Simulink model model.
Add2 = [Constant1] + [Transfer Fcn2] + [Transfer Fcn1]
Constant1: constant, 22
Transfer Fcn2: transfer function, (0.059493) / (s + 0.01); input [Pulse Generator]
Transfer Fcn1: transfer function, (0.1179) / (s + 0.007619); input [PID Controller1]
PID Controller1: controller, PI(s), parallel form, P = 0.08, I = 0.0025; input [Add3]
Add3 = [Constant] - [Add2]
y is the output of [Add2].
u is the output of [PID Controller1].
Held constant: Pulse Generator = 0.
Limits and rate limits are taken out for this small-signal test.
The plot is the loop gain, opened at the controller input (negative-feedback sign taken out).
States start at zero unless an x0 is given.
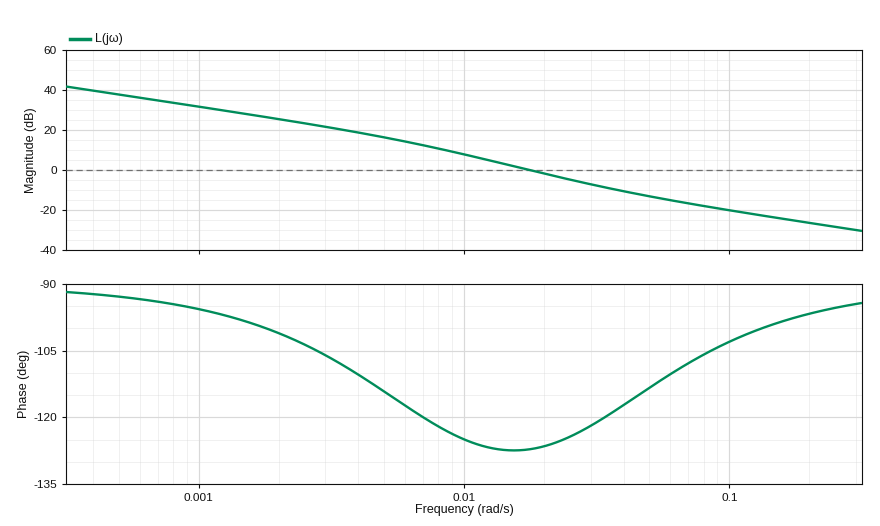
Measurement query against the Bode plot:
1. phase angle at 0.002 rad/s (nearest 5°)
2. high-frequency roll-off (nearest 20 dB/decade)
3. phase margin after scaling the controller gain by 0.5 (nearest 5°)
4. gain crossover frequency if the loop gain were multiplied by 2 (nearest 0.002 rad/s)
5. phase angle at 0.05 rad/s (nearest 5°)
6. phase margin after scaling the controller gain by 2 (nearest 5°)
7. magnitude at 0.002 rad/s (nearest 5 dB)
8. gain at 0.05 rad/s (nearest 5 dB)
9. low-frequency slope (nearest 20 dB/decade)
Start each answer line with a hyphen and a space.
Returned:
- -100°
- -20 dB/decade
- 55°
- 0.028 rad/s
- -115°
- 55°
- 25 dB
- -15 dB
- -20 dB/decade
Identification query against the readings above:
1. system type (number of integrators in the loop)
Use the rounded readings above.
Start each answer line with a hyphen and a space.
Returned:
- 1
